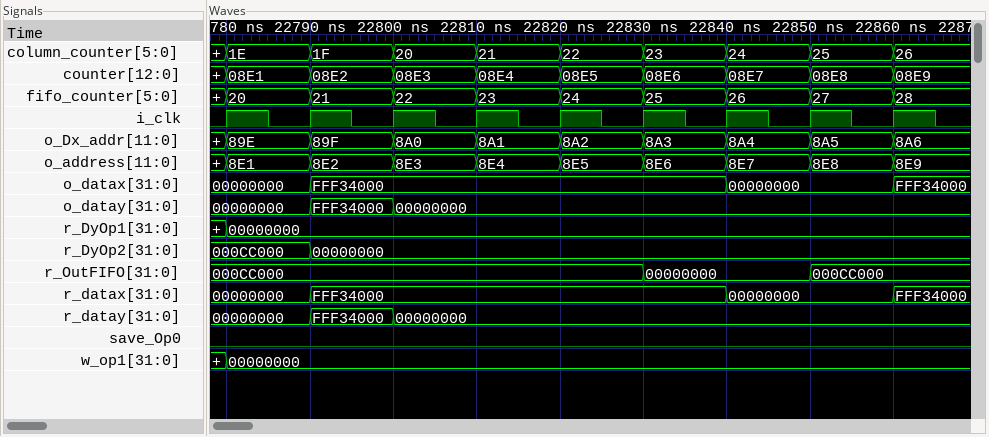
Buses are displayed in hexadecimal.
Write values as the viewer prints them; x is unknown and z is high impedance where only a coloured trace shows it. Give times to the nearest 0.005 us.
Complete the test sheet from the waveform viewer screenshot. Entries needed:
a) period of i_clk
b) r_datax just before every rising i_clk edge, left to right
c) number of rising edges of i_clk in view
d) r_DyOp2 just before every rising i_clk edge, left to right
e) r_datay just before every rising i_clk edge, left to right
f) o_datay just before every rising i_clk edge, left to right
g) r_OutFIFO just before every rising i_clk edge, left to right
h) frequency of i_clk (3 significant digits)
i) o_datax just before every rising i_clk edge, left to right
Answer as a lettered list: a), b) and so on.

a) 0.01 us
b) 00000000, 00000000, FFF34000, FFF34000, FFF34000, FFF34000, FFF34000, 00000000, 00000000
c) 9
d) 000CC000, 000CC000, 00000000, 00000000, 00000000, 00000000, 00000000, 00000000, 00000000
e) 00000000, 00000000, FFF34000, 00000000, 00000000, 00000000, 00000000, 00000000, 00000000
f) 00000000, 00000000, FFF34000, 00000000, 00000000, 00000000, 00000000, 00000000, 00000000
g) 000CC000, 000CC000, 000CC000, 000CC000, 000CC000, 000CC000, 00000000, 00000000, 000CC000
h) 100 MHz
i) 00000000, 00000000, FFF34000, FFF34000, FFF34000, FFF34000, FFF34000, 00000000, 00000000
